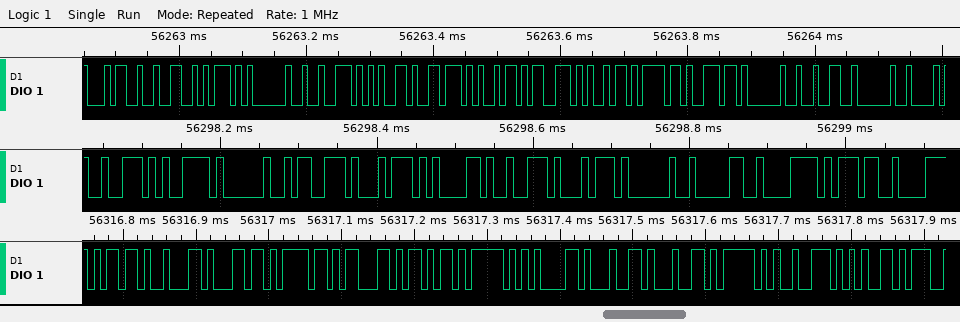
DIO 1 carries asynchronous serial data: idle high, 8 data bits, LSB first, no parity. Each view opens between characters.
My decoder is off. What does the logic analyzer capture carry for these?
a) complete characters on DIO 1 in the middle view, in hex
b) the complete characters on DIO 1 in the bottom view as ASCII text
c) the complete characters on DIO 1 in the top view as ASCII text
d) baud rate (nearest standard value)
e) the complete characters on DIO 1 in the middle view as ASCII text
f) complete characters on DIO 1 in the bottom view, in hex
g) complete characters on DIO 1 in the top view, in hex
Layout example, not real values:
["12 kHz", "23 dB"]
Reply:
["72, 79, 20, 73, 74, 61, 72, 74, 20, 30, 78, 37", "\"mblock_add_re\"", "\"42] revision 2 \"", "115200 baud", "\"ry start 0x7\"", "6D, 62, 6C, 6F, 63, 6B, 5F, 61, 64, 64, 5F, 72, 65", "34, 32, 5D, 20, 72, 65, 76, 69, 73, 69, 6F, 6E, 20, 32, 20"]
